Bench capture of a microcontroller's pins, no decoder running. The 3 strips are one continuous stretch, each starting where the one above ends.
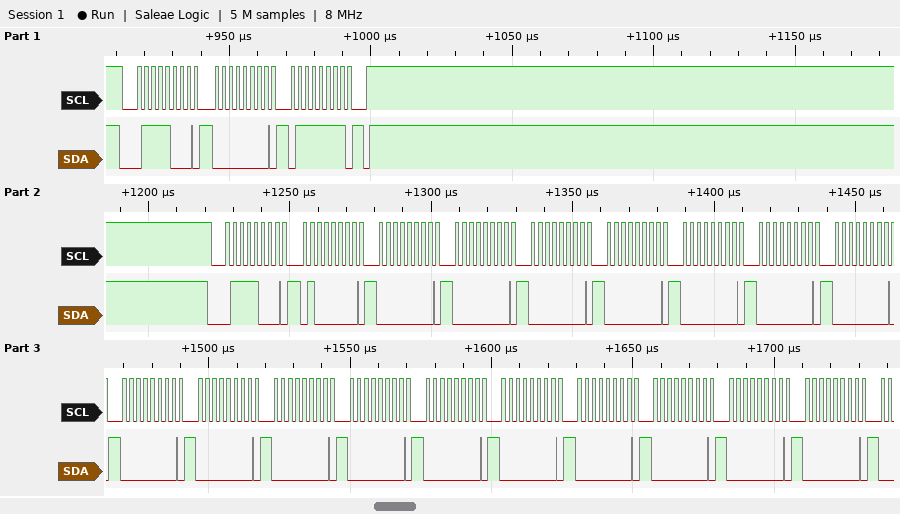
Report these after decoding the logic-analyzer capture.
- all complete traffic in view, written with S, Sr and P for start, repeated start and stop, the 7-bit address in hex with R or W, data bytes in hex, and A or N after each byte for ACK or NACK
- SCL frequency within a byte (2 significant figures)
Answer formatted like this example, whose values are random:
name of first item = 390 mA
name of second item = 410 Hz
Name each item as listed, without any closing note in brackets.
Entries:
all complete traffic in view, written with S, Sr and P for start, repeated start and stop, the 7-bit address in hex with R or W, data bytes in hex, and A or N after each byte for ACK or NACK = S 3CW A 00 A 7F A P S 3CW A 40 A 00 A 00 A 00 A 00 A 00 A 00 A 00 A 00 A 00 A 00 A 00 A 00 A 00 A 00 A 00 A 00 A 00 A
SCL frequency within a byte = 400 kHz
